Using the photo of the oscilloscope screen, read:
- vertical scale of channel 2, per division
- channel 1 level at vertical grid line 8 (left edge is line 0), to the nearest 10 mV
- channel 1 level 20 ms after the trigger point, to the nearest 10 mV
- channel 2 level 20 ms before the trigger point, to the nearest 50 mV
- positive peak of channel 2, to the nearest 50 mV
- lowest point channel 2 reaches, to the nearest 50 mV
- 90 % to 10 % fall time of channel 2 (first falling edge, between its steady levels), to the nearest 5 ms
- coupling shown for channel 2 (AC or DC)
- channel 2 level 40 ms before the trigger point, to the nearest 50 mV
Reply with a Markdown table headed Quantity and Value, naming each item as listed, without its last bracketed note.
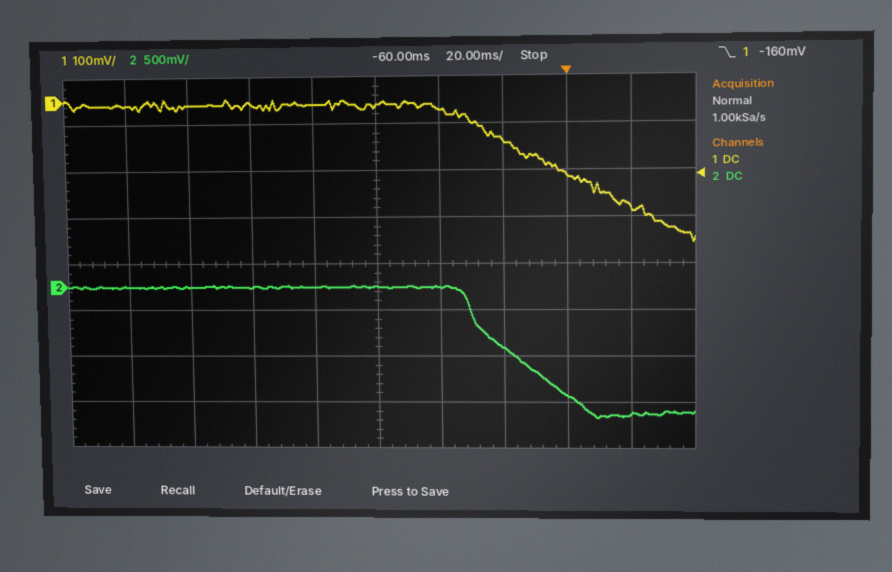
| Quantity | Value |
|---|---|
| vertical scale of channel 2, per division | 500 mV |
| channel 1 level at vertical grid line 8 (left edge is line 0), to the nearest 10 mV | -160 mV |
| channel 1 level 20 ms after the trigger point, to the nearest 10 mV | -230 mV |
| channel 2 level 20 ms before the trigger point, to the nearest 50 mV | -650 mV |
| positive peak of channel 2, to the nearest 50 mV | 0 mV |
| lowest point channel 2 reaches, to the nearest 50 mV | -1.40 V |
| 90 % to 10 % fall time of channel 2 (first falling edge, between its steady levels), to the nearest 5 ms | 35 ms |
| coupling shown for channel 2 | DC |
| channel 2 level 40 ms before the trigger point, to the nearest 50 mV | 0 mV |
